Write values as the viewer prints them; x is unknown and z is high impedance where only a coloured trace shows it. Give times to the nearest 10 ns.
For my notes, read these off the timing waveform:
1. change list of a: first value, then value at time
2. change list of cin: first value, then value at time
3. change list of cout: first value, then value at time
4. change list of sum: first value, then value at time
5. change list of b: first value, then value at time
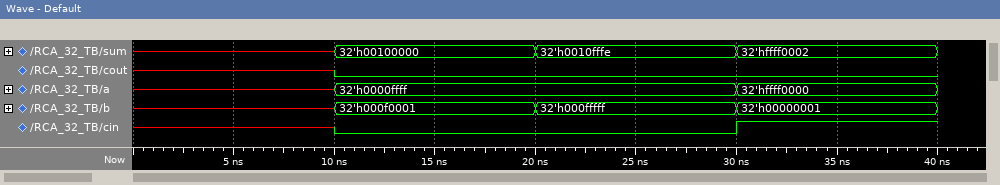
x, 32'h0000ffff at 10 ns, 32'hffff0000 at 30 ns
x, 0 at 10 ns, 1 at 30 ns
x, 0 at 10 ns
x, 32'h00100000 at 10 ns, 32'h0010fffe at 20 ns, 32'hffff0002 at 30 ns
x, 32'h000f0001 at 10 ns, 32'h000fffff at 20 ns, 32'h00000001 at 30 ns
